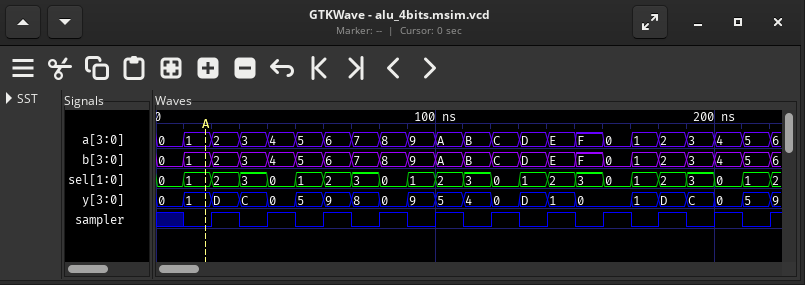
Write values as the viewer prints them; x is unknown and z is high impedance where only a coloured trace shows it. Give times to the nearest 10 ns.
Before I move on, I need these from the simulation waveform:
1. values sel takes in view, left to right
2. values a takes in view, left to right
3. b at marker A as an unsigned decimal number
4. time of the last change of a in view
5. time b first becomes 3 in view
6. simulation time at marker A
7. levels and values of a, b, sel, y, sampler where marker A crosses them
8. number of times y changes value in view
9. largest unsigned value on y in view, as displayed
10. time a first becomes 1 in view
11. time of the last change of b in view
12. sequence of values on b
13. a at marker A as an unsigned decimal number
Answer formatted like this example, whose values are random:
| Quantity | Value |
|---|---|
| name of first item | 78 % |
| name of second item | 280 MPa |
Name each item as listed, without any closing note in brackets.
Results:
| Quantity | Value |
|---|---|
| values sel takes in view, left to right | 0, 1, 2, 3, 0, 1, 2, 3, 0, 1, 2, 3, 0, 1, 2, 3, 0, 1, 2, 3, 0, 1, 2 |
| values a takes in view, left to right | 0, 1, 2, 3, 4, 5, 6, 7, 8, 9, A, B, C, D, E, F, 0, 1, 2, 3, 4, 5, 6 |
| b at marker A as an unsigned decimal number | 1 |
| time of the last change of a in view | 220 ns |
| time b first becomes 3 in view | 30 ns |
| simulation time at marker A | 20 ns |
| levels and values of a, b, sel, y, sampler where marker A crosses them | a=1, b=1, sel=1, y=1, sampler=0 |
| number of times y changes value in view | 21 |
| largest unsigned value on y in view, as displayed | D |
| time a first becomes 1 in view | 10 ns |
| time of the last change of b in view | 220 ns |
| sequence of values on b | 0, 1, 2, 3, 4, 5, 6, 7, 8, 9, A, B, C, D, E, F, 0, 1, 2, 3, 4, 5, 6 |
| a at marker A as an unsigned decimal number | 1 |
